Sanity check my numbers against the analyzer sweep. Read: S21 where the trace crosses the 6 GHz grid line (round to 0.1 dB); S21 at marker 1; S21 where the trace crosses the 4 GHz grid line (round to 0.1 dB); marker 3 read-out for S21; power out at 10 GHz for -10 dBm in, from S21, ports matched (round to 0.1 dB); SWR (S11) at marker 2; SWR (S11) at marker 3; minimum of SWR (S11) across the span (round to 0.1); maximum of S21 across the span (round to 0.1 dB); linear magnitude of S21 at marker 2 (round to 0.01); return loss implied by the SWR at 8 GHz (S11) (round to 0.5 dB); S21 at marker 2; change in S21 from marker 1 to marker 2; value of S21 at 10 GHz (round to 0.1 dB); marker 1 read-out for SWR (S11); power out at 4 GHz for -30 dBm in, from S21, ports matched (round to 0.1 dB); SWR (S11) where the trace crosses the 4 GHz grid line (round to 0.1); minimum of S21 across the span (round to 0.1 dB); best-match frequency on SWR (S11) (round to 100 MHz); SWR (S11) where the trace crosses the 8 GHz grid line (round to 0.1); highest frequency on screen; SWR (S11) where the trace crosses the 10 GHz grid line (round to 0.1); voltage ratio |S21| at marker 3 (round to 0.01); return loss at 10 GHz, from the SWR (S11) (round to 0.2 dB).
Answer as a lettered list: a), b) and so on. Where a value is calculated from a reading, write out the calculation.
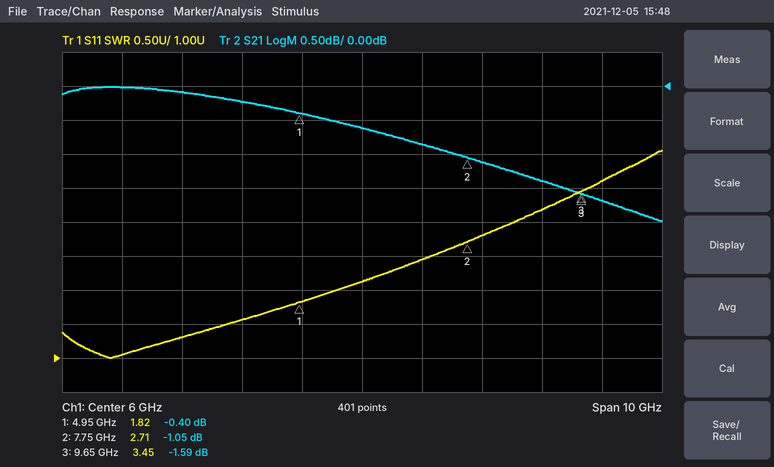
a) -0.6 dB
b) -0.40 dB
c) -0.2 dB
d) -1.59 dB
e) -10 dBm + (-1.7 dB) = -11.7 dBm
f) 2.71
g) 3.45
h) 1.0
i) 0.0 dB
j) 10^(-1.05/20) ≈ 0.89
k) −20 log10((2.8 − 1)/(2.8 + 1)) ≈ 6.5 dB
l) -1.05 dB
m) -1.05 − (-0.4) = -0.65 dB
n) -1.7 dB
o) 1.82
p) -30 dBm + (-0.2 dB) = -30.2 dBm
q) 1.6
r) -2.0 dB
s) 1.8 GHz
t) 2.8
u) 11 GHz
v) 3.6
w) 10^(-1.59/20) ≈ 0.83
x) −20 log10((3.6 − 1)/(3.6 + 1)) ≈ 5.0 dB
